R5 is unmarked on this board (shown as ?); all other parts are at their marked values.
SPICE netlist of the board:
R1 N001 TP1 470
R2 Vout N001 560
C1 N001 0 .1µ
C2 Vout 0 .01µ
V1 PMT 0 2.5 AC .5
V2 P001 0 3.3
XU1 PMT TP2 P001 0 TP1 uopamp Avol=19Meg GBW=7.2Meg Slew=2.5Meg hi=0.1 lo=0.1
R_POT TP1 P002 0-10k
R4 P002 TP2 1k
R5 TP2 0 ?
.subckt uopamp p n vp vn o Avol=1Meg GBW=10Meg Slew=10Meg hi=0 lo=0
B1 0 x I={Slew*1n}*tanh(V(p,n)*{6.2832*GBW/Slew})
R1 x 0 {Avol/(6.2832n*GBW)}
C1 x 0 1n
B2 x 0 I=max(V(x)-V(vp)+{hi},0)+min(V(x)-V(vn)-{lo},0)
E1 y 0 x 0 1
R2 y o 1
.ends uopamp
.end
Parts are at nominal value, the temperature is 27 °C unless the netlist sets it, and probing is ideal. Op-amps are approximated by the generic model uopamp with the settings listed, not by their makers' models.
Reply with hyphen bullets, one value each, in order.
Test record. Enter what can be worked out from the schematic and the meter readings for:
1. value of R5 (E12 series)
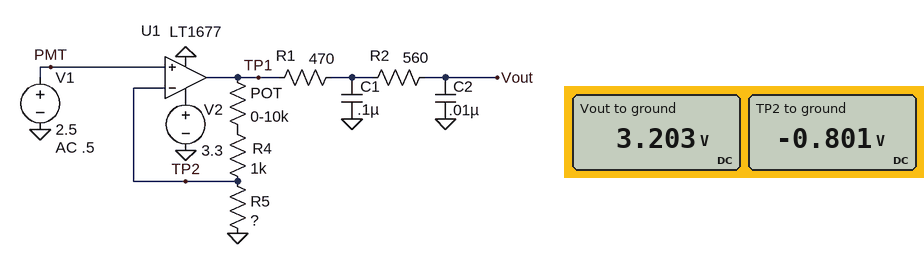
- 1.8 kΩ
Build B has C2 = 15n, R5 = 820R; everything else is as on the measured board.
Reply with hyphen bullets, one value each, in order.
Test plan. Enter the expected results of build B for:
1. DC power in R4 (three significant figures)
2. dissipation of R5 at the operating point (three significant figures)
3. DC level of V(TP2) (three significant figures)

- 153 µW
- 126 µW
- -321 mV
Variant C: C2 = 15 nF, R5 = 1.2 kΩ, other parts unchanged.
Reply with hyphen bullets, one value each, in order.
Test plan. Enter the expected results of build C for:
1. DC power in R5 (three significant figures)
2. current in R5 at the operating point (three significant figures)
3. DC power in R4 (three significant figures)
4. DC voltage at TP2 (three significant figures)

- 202 µW
- 411 µA
- 169 µW
- -493 mV
